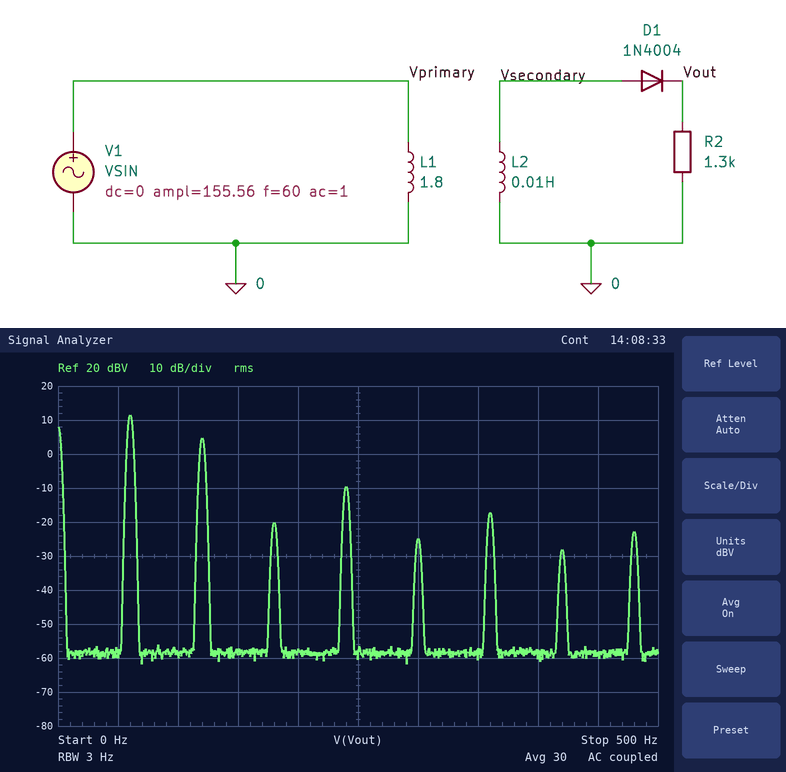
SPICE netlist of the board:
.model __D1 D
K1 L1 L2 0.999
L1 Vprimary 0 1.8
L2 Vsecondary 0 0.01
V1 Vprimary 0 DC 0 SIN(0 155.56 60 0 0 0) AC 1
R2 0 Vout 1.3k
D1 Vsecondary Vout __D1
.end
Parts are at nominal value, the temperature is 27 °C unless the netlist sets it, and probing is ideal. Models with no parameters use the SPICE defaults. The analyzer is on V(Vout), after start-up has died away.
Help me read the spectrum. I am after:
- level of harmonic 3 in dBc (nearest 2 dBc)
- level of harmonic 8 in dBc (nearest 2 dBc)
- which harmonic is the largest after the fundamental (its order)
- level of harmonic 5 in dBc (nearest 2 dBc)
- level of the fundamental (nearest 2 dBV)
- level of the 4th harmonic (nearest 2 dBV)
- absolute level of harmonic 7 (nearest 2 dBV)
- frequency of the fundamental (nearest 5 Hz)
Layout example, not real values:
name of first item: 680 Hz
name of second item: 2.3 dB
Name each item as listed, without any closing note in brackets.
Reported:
level of harmonic 3 in dBc: -32 dBc
level of harmonic 8 in dBc: -34 dBc
which harmonic is the largest after the fundamental: 2
level of harmonic 5 in dBc: -36 dBc
level of the fundamental: 12 dBV
level of the 4th harmonic: -10 dBV
absolute level of harmonic 7: -28 dBV
frequency of the fundamental: 60 Hz
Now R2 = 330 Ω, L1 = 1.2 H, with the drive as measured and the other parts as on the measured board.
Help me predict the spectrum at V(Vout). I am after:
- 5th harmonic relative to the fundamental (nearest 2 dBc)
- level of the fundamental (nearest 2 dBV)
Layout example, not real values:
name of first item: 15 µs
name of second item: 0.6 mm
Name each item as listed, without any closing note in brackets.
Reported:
5th harmonic relative to the fundamental: -38 dBc
level of the fundamental: 14 dBV
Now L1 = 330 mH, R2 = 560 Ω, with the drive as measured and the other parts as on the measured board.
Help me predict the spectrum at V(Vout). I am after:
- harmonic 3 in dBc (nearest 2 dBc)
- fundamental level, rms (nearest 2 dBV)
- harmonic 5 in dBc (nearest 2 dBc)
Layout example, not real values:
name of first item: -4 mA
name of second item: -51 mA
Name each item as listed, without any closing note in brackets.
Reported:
harmonic 3 in dBc: -38 dBc
fundamental level, rms: 20 dBV
harmonic 5 in dBc: -44 dBc
